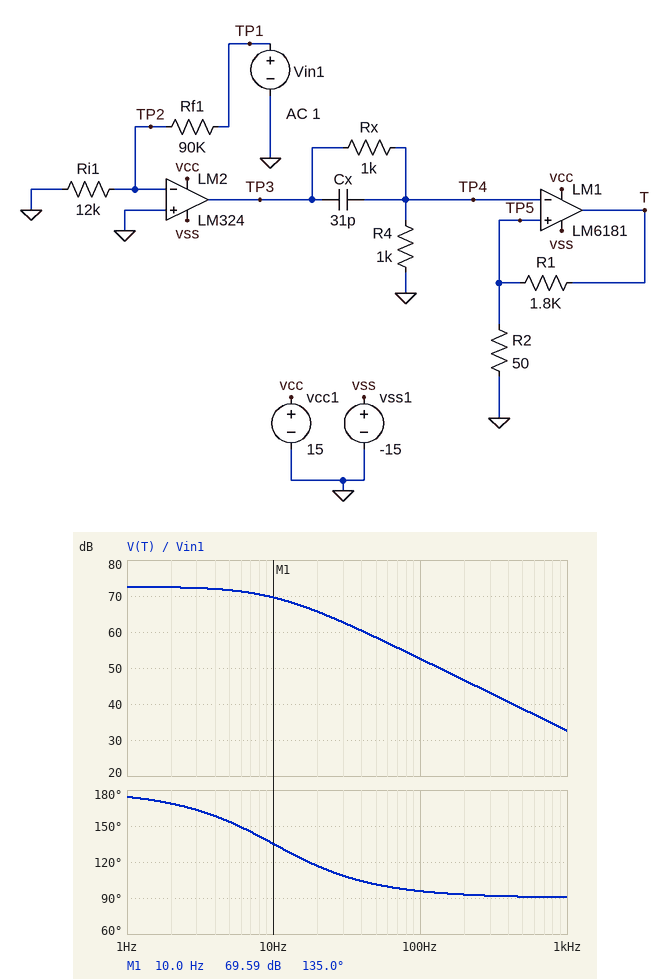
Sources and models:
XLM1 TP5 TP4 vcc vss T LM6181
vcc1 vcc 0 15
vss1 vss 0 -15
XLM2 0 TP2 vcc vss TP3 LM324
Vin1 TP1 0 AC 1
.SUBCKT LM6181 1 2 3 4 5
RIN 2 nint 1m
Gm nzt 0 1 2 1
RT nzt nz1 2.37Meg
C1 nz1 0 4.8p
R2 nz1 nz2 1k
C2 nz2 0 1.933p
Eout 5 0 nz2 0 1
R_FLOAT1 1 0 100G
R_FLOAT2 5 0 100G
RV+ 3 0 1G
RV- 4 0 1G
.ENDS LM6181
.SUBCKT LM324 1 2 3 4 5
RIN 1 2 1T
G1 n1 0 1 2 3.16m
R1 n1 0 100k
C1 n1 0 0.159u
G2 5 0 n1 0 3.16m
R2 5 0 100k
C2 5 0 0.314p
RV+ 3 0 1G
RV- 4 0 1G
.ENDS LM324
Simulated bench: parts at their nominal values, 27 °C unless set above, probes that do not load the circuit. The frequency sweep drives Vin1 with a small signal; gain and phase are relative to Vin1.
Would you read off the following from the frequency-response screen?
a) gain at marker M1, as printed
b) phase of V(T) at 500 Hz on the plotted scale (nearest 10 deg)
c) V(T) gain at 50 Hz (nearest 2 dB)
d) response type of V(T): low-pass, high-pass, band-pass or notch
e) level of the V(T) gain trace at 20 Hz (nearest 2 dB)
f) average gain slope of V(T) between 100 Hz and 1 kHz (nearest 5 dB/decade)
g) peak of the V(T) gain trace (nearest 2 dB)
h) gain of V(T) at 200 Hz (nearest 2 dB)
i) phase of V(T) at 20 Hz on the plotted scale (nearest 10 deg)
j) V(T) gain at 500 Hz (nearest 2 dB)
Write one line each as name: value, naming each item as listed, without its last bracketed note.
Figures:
gain at marker M1, as printed: 69.59 dB
phase of V(T) at 500 Hz on the plotted scale: 90 deg
V(T) gain at 50 Hz: 58 dB
response type of V(T): low-pass, high-pass, band-pass or notch: low-pass
level of the V(T) gain trace at 20 Hz: 66 dB
average gain slope of V(T) between 100 Hz and 1 kHz: -20 dB/decade
peak of the V(T) gain trace: 72 dB
gain of V(T) at 200 Hz: 46 dB
phase of V(T) at 20 Hz on the plotted scale: 120 deg
V(T) gain at 500 Hz: 38 dB
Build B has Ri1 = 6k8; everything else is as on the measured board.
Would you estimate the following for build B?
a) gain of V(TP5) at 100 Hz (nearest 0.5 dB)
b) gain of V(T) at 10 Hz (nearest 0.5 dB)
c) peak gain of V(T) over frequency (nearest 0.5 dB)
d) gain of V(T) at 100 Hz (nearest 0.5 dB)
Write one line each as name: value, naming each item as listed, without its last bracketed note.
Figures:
gain of V(TP5) at 100 Hz: 16.5 dB
gain of V(T) at 10 Hz: 65.0 dB
peak gain of V(T) over frequency: 68.0 dB
gain of V(T) at 100 Hz: 48.0 dB
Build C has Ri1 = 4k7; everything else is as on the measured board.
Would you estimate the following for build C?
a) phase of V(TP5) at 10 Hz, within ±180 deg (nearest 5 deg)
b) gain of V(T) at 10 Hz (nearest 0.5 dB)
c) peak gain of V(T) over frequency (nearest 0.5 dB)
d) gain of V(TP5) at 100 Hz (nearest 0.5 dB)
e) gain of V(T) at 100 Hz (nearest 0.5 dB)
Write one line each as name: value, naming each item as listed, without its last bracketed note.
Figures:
phase of V(TP5) at 10 Hz, within ±180 deg: 135 deg
gain of V(T) at 10 Hz: 62.0 dB
peak gain of V(T) over frequency: 65.0 dB
gain of V(TP5) at 100 Hz: 13.5 dB
gain of V(T) at 100 Hz: 45.0 dB
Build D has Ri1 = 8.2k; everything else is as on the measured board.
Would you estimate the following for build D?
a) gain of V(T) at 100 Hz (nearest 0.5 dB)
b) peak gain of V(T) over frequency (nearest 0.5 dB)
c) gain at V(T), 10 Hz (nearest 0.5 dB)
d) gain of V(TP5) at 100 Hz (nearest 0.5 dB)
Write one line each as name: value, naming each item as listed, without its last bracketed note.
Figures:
gain of V(T) at 100 Hz: 49.5 dB
peak gain of V(T) over frequency: 69.5 dB
gain at V(T), 10 Hz: 66.5 dB
gain of V(TP5) at 100 Hz: 18.0 dB
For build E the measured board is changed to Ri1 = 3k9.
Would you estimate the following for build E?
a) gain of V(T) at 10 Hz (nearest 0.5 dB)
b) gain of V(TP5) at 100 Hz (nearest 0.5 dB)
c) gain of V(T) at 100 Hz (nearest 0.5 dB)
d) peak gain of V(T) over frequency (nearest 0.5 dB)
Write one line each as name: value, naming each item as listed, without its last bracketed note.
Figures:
gain of V(T) at 10 Hz: 60.5 dB
gain of V(TP5) at 100 Hz: 12.0 dB
gain of V(T) at 100 Hz: 43.5 dB
peak gain of V(T) over frequency: 63.5 dB
